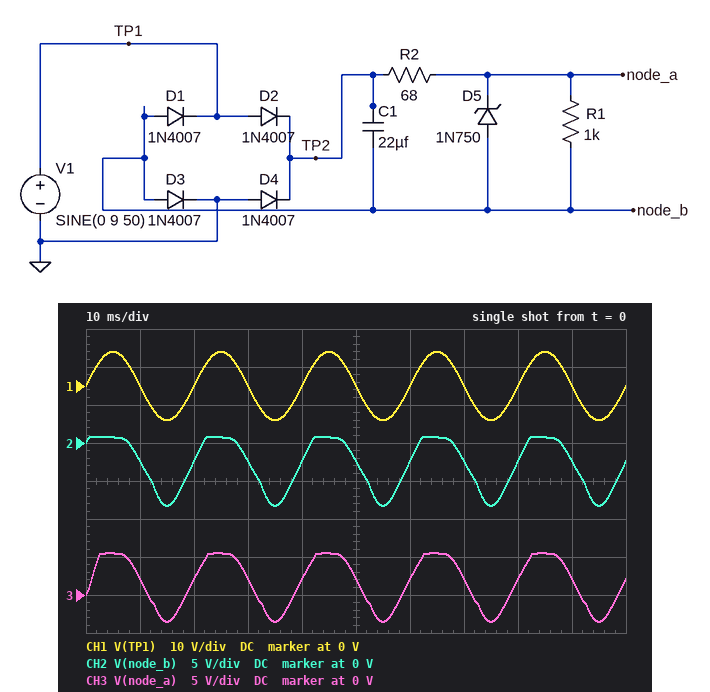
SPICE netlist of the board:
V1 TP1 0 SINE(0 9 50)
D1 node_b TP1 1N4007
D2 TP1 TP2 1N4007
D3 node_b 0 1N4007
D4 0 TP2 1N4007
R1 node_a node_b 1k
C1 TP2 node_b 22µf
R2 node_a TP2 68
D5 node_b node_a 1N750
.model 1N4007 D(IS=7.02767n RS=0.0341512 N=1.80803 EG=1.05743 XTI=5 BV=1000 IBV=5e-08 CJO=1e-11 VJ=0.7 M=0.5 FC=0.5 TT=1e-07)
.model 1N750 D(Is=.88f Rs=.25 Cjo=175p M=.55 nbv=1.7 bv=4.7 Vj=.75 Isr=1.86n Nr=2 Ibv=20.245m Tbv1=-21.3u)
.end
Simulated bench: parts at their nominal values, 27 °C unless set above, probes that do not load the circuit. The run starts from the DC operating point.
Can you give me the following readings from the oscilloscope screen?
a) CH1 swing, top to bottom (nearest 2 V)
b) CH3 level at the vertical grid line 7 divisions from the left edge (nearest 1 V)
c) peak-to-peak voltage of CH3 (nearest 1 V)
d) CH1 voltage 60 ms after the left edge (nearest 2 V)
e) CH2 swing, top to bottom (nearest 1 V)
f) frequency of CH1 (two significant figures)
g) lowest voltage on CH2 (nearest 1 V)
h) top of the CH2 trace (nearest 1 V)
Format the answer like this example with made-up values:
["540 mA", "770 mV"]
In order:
["18 V", "2 V", "9 V", "0 V", "9 V", "50 Hz", "-8 V", "1 V"]
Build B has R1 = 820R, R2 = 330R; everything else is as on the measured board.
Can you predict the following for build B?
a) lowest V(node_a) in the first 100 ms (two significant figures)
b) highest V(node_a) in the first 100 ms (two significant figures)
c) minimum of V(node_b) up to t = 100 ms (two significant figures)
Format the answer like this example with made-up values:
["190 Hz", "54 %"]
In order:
["-3.7 V", "5.3 V", "-8.3 V"]
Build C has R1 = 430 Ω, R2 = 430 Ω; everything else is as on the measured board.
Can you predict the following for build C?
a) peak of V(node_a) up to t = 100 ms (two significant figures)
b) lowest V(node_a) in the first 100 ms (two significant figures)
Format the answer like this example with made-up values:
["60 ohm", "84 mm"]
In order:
["4.5 V", "-4.5 V"]
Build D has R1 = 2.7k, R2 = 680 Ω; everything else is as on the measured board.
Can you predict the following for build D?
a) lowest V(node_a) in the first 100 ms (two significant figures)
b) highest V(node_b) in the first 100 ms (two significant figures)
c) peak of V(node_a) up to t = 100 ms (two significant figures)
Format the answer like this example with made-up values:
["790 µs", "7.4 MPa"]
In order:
["-3.7 V", "750 mV", "5.3 V"]
